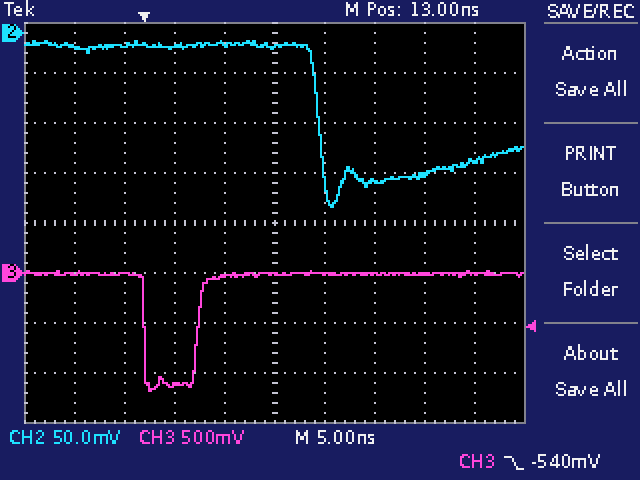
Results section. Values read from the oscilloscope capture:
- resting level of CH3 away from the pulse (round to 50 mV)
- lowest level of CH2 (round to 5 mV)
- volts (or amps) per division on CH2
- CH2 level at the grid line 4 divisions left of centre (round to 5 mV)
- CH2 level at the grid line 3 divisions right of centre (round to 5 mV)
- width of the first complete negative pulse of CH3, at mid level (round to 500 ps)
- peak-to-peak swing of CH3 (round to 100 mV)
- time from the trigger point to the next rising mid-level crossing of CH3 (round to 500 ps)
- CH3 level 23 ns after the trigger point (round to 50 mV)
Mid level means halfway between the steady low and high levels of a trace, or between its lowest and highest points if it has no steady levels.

0 mV
-175 mV
50 mV
-15 mV
-140 mV
5.5 ns
1.20 V
5.5 ns
0 mV
